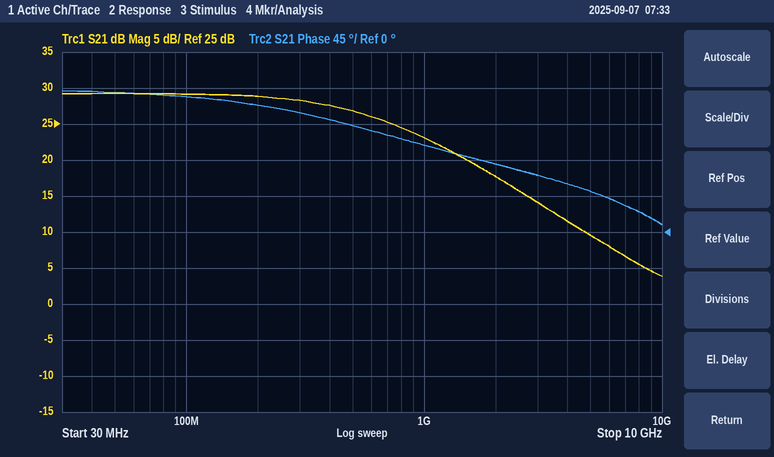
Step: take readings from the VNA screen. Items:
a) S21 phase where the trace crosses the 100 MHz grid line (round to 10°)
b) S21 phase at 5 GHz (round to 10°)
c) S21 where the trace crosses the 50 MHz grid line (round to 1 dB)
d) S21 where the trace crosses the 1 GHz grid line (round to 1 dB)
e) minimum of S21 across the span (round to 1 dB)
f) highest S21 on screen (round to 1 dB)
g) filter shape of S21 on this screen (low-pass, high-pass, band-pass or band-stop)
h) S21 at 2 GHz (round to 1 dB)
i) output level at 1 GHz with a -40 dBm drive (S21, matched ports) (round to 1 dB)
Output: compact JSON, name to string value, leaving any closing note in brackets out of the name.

{"S21 phase where the trace crosses the 100 MHz grid line": "170°", "S21 phase at 5 GHz": "50°", "S21 where the trace crosses the 50 MHz grid line": "29 dB", "S21 where the trace crosses the 1 GHz grid line": "23 dB", "minimum of S21 across the span": "4 dB", "highest S21 on screen": "29 dB", "filter shape of S21 on this screen": "low-pass", "S21 at 2 GHz": "18 dB", "output level at 1 GHz with a -40 dBm drive (S21, matched ports)": "-17 dBm"}
